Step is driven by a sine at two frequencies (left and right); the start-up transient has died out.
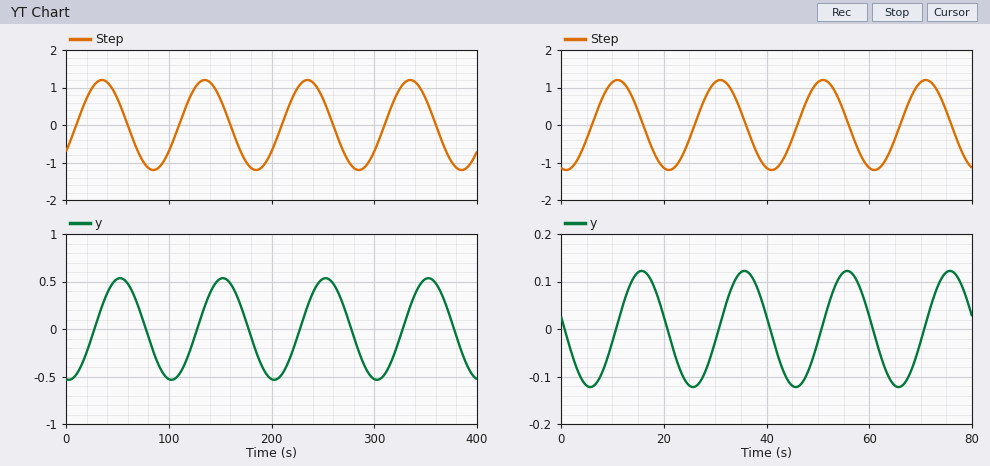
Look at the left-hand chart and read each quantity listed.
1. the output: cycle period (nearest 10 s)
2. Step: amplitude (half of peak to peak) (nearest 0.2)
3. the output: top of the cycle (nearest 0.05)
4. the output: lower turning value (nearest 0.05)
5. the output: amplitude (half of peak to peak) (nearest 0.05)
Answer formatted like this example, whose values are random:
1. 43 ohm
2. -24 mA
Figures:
1. 100 s
2. 1.2
3. 0.55
4. -0.55
5. 0.55
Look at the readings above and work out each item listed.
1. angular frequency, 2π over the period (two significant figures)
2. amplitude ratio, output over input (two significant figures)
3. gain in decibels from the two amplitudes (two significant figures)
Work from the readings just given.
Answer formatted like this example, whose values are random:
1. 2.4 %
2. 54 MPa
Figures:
1. 0.063 rad/s
2. 0.46
3. -6.8 dB
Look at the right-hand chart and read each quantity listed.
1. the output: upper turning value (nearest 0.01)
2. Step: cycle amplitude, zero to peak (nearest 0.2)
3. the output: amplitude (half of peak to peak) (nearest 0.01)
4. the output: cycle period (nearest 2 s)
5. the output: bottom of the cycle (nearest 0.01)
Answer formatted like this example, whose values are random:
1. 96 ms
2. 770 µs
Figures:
1. 0.12
2. 1.2
3. 0.12
4. 20 s
5. -0.12
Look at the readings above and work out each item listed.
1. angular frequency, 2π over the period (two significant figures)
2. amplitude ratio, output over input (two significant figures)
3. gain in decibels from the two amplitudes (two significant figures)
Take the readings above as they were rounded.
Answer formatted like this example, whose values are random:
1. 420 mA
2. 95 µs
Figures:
1. 0.31 rad/s
2. 0.10
3. -20 dB
